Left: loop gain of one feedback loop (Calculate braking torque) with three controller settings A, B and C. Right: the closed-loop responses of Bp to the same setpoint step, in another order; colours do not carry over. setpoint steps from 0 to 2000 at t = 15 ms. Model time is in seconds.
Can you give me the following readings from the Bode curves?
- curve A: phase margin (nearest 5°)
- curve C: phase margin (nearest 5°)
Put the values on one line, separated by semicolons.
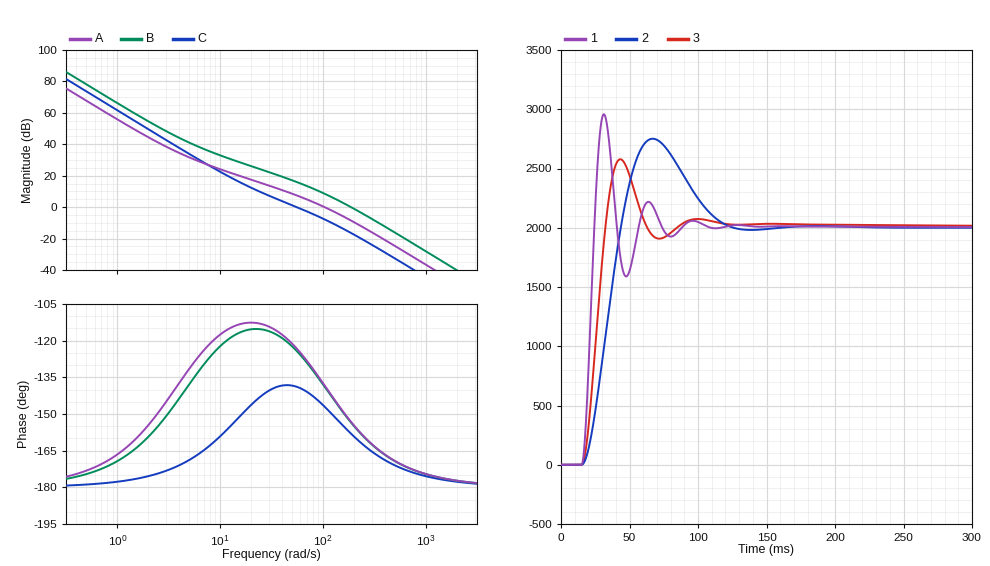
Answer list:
40°; 40°
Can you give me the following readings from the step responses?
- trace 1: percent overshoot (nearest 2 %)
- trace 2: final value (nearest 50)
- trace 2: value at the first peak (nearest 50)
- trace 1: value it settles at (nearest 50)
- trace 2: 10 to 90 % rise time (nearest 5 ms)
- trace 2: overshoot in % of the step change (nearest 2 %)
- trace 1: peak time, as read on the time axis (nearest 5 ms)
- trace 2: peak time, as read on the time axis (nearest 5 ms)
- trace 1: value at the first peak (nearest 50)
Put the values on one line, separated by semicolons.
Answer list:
48 %; 2000; 2750; 2000; 20 ms; 38 %; 30 ms; 65 ms; 2950
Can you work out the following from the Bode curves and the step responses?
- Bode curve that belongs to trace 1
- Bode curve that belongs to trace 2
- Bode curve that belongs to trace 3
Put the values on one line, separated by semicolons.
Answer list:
B; C; A
